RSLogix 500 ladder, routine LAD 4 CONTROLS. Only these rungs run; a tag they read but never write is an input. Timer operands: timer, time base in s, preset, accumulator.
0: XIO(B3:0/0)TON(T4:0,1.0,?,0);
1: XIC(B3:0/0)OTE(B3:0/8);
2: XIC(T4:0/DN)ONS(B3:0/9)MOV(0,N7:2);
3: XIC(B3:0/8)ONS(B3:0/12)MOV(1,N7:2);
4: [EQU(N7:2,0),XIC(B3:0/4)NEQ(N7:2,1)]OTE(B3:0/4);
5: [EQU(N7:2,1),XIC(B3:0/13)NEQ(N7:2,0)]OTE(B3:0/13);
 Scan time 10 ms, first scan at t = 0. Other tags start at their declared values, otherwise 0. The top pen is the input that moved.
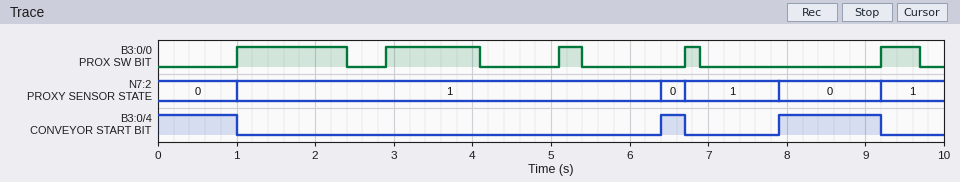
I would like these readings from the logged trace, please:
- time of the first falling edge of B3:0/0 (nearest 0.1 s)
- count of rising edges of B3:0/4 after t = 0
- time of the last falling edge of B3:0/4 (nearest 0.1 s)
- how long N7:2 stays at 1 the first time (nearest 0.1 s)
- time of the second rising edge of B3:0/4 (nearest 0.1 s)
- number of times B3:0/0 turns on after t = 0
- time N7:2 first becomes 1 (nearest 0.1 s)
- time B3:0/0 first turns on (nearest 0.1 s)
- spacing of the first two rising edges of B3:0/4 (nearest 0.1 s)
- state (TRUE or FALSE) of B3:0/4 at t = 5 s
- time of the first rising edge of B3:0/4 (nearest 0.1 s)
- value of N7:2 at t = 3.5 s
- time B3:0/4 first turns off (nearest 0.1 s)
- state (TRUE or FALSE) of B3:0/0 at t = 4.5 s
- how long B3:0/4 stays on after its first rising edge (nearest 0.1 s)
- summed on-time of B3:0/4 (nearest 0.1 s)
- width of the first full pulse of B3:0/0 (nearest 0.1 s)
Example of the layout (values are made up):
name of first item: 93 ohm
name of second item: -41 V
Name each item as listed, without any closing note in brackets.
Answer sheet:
time of the first falling edge of B3:0/0: 2.4 s
count of rising edges of B3:0/4 after t = 0: 2
time of the last falling edge of B3:0/4: 9.2 s
how long N7:2 stays at 1 the first time: 5.4 s
time of the second rising edge of B3:0/4: 7.9 s
number of times B3:0/0 turns on after t = 0: 5
time N7:2 first becomes 1: 1.0 s
time B3:0/0 first turns on: 1.0 s
spacing of the first two rising edges of B3:0/4: 1.5 s
state (TRUE or FALSE) of B3:0/4 at t = 5 s: FALSE
time of the first rising edge of B3:0/4: 6.4 s
value of N7:2 at t = 3.5 s: 1
time B3:0/4 first turns off: 1.0 s
state (TRUE or FALSE) of B3:0/0 at t = 4.5 s: FALSE
how long B3:0/4 stays on after its first rising edge: 0.3 s
summed on-time of B3:0/4: 2.6 s
width of the first full pulse of B3:0/0: 1.4 s
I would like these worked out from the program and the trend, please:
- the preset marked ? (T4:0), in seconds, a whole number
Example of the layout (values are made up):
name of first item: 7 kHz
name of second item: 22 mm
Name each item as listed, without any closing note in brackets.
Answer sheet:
the preset marked ? (T4:0), in seconds, a whole number: 1 s
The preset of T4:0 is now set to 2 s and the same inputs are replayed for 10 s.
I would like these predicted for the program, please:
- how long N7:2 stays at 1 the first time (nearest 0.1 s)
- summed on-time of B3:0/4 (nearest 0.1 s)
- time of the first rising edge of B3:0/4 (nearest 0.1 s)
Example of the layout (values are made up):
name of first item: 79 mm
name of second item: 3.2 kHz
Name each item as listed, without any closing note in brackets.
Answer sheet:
how long N7:2 stays at 1 the first time: 7.9 s
summed on-time of B3:0/4: 1.3 s
time of the first rising edge of B3:0/4: 8.9 s
